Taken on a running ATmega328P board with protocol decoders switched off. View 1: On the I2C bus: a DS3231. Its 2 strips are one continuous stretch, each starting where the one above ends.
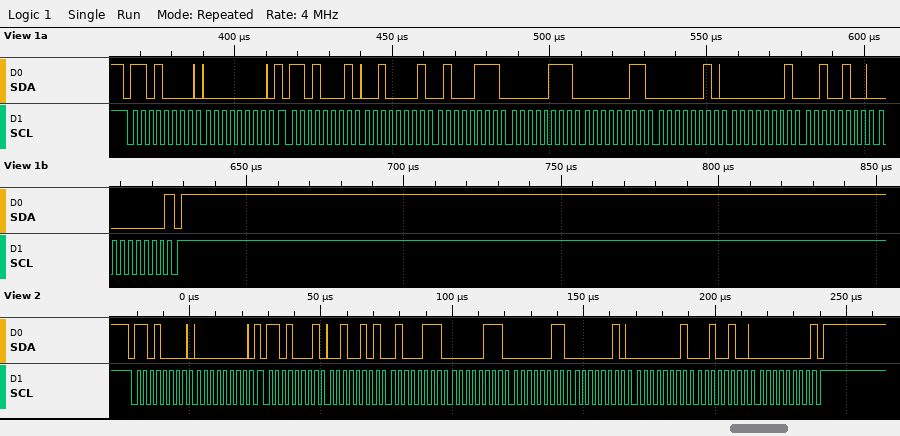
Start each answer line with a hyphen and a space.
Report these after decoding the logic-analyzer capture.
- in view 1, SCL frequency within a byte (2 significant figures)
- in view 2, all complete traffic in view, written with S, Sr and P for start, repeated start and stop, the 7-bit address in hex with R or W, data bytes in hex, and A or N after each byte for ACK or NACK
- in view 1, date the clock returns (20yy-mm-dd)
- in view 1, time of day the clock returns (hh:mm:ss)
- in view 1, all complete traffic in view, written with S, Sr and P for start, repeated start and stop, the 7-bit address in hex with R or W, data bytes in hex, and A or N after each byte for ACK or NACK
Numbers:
- 400 kHz
- S 68W A 00 A Sr 68R A 25 A 47 A 07 A 03 A 02 A 01 A 24 A 00 N P
- 2024-01-02
- 07:47:21
- S 68W A 00 A Sr 68R A 21 A 47 A 07 A 03 A 02 A 01 A 24 A 00 N P
